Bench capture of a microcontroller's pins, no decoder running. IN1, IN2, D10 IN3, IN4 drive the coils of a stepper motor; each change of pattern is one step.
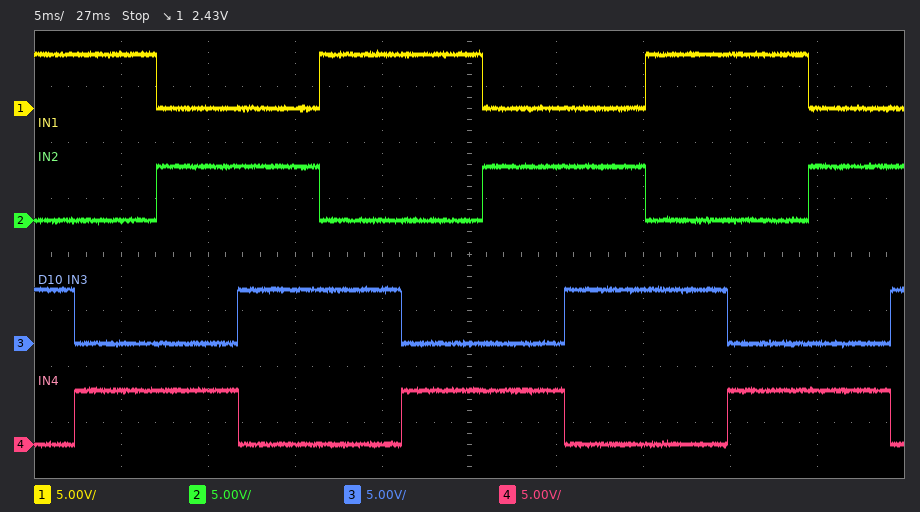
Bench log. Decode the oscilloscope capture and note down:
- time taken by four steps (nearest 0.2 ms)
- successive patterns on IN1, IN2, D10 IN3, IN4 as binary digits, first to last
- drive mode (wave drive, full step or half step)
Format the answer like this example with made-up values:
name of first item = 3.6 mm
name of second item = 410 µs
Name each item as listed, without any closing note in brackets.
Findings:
time taken by four steps = 18.8 ms
successive patterns on IN1, IN2, D10 IN3, IN4 as binary digits, first to last = 1010 1001 0101 0110 1010 1001 0101 0110 1010 1001 0101 0110
drive mode = full step
